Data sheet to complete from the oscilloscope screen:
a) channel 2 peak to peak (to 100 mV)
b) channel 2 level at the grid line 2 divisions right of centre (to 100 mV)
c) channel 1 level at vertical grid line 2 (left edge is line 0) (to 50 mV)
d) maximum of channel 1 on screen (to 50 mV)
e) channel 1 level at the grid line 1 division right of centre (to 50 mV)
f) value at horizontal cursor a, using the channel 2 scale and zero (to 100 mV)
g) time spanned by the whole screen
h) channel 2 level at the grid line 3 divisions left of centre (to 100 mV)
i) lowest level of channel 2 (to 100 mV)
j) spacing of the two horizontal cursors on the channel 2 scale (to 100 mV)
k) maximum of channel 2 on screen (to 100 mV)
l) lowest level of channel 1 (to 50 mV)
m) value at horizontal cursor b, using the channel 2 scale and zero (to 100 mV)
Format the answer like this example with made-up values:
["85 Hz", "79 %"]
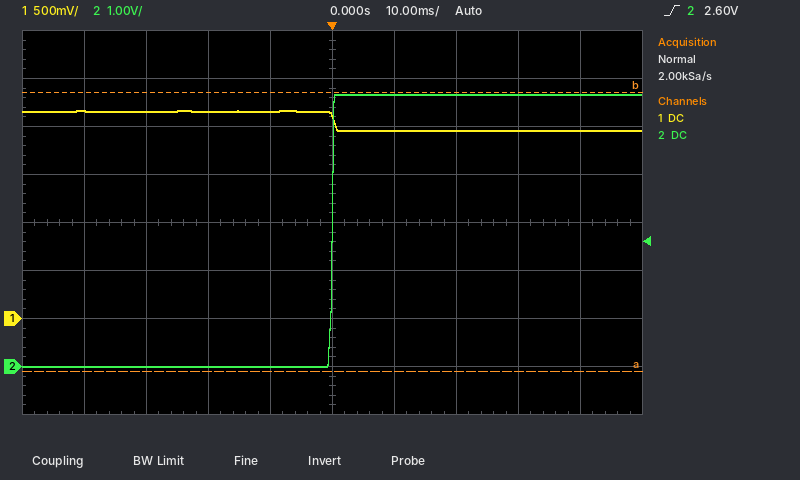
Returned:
["5.7 V", "5.7 V", "2.15 V", "2.15 V", "1.95 V", "-100 mV", "100 ms", "0.0 V", "0.0 V", "5.8 V", "5.7 V", "1.95 V", "5.7 V"]
